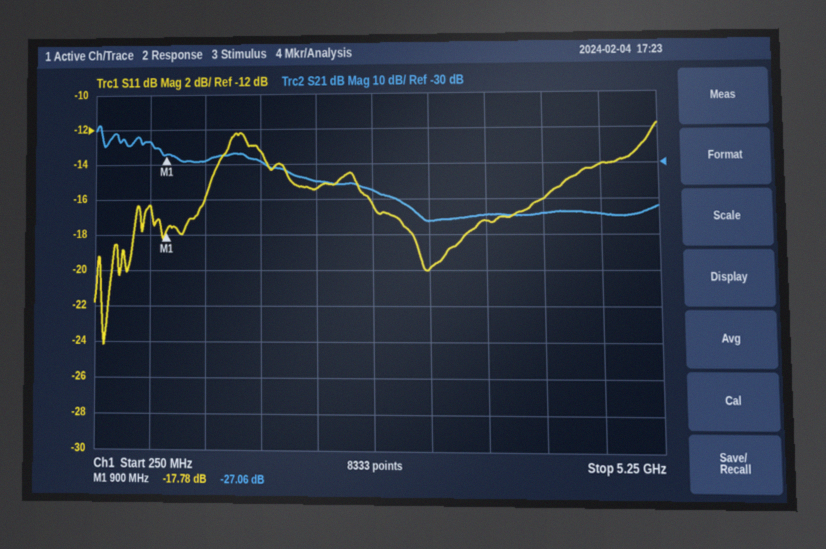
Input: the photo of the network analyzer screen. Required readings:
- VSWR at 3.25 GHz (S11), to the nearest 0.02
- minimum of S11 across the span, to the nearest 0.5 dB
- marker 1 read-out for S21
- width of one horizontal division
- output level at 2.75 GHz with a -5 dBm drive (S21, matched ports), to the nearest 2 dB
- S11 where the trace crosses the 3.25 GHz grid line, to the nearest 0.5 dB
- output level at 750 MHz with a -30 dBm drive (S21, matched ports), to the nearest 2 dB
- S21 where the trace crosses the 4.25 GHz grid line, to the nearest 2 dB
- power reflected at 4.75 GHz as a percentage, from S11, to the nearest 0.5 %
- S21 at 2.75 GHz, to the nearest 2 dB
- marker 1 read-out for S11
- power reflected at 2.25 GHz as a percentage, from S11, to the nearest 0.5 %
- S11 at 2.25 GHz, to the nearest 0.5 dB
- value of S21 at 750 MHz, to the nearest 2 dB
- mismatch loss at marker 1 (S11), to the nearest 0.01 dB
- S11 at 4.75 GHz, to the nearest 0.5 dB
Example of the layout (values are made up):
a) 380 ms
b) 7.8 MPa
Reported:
a) 1.22
b) -24.0 dB
c) -27.06 dB
d) 500 MHz
e) -42 dBm
f) -20.0 dB
g) -54 dBm
h) -44 dB
i) 4.0 %
j) -38 dB
k) -17.78 dB
l) 3.0 %
m) -15.5 dB
n) -24 dB
o) 0.07 dB
p) -14.0 dB
